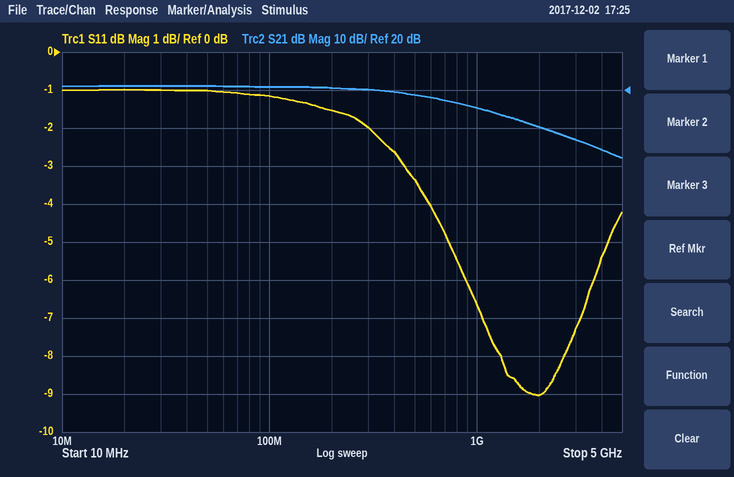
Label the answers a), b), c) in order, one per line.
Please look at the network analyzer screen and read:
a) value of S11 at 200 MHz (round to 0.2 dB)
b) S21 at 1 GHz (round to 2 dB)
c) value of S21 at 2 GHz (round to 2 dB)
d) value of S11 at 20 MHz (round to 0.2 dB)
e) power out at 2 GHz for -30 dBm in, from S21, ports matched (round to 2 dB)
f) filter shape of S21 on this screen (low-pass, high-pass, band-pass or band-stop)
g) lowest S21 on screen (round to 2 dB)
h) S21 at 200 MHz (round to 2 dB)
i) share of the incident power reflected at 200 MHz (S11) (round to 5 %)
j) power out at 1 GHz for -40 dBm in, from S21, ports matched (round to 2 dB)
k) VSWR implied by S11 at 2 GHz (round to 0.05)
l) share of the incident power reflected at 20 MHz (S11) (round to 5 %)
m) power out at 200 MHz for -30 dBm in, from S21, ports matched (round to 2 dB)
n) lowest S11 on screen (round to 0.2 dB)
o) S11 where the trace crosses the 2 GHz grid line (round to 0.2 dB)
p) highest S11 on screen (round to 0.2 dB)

a) -1.6 dB
b) 16 dB
c) 10 dB
d) -1.0 dB
e) -20 dBm
f) low-pass
g) 2 dB
h) 20 dB
i) 70 %
j) -24 dBm
k) 2.10
l) 80 %
m) -10 dBm
n) -9.0 dB
o) -9.0 dB
p) -1.0 dB
